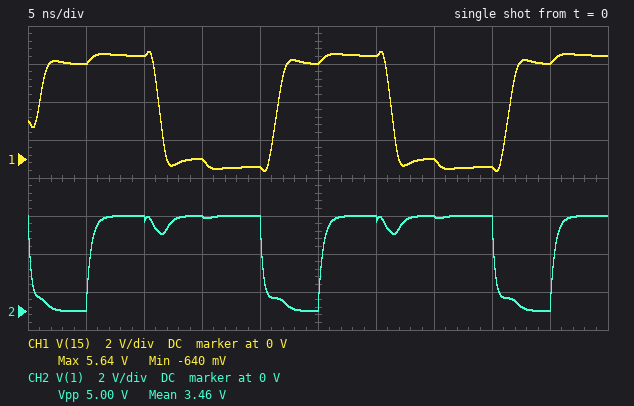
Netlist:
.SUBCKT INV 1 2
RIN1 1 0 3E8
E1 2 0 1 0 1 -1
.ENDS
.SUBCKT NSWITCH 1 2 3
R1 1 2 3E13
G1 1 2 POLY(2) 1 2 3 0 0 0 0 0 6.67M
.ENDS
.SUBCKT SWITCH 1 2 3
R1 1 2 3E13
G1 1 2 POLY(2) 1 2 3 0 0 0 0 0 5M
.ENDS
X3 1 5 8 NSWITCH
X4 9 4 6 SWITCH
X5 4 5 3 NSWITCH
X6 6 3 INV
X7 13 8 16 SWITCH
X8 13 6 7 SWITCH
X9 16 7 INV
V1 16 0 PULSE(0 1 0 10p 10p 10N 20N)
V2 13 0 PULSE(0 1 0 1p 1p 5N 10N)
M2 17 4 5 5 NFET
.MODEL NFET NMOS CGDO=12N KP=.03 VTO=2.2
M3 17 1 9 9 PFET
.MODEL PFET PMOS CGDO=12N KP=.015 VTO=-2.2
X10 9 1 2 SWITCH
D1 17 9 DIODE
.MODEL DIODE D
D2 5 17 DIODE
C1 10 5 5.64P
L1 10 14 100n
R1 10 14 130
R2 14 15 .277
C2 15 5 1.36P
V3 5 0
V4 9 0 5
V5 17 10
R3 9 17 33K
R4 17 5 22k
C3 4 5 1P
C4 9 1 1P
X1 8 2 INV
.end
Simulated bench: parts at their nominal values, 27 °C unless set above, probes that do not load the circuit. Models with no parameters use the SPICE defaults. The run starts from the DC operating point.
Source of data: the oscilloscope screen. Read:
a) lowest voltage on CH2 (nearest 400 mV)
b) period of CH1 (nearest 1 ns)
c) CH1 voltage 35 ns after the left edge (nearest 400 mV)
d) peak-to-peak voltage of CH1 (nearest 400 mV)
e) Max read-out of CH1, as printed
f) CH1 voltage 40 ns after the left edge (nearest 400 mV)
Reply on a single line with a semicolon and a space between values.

0 V; 20 ns; 0 V; 6.4 V; 5.64 V; -400 mV
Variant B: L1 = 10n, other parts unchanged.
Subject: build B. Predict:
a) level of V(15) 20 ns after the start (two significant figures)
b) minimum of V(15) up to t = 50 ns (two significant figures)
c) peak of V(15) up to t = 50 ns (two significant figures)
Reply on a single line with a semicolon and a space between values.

-420 mV; -770 mV; 5.8 V
